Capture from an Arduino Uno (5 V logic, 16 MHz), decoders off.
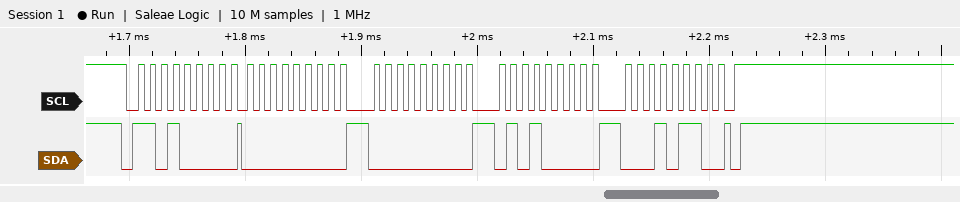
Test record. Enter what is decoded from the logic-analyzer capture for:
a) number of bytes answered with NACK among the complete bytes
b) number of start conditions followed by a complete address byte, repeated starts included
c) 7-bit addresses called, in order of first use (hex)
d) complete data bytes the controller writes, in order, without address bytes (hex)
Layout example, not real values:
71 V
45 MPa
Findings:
0
1
0x68
00 00 50 16
